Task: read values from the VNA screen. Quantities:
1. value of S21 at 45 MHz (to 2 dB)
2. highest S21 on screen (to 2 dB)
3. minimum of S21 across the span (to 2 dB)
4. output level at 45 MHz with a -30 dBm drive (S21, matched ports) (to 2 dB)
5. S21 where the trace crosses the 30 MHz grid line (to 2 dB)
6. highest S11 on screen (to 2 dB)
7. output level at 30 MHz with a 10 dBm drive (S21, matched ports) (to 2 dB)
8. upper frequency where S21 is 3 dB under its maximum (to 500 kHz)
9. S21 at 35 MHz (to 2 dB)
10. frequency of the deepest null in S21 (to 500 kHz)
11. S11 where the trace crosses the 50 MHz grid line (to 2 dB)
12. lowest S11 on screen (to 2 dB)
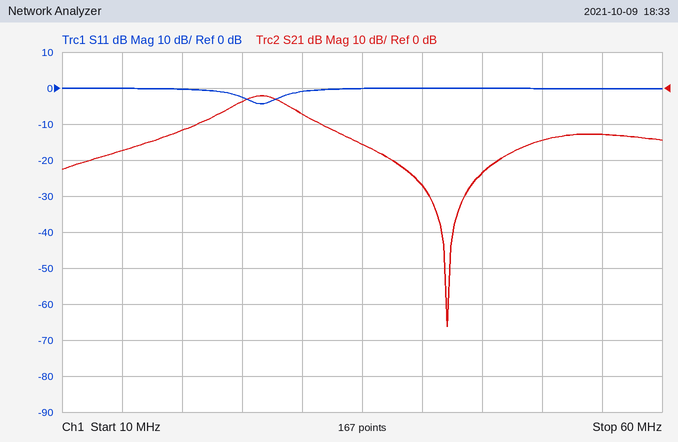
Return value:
-24 dB
-2 dB
-66 dB
-54 dBm
-8 dB
0 dB
2 dBm
29.0 MHz
-16 dB
42.0 MHz
0 dB
-4 dB
